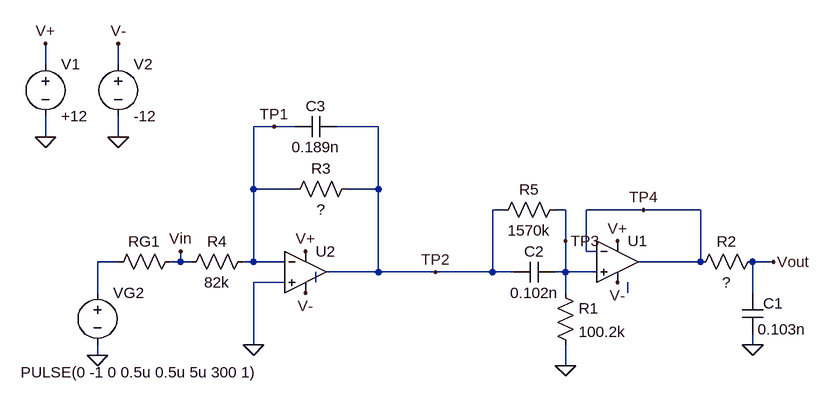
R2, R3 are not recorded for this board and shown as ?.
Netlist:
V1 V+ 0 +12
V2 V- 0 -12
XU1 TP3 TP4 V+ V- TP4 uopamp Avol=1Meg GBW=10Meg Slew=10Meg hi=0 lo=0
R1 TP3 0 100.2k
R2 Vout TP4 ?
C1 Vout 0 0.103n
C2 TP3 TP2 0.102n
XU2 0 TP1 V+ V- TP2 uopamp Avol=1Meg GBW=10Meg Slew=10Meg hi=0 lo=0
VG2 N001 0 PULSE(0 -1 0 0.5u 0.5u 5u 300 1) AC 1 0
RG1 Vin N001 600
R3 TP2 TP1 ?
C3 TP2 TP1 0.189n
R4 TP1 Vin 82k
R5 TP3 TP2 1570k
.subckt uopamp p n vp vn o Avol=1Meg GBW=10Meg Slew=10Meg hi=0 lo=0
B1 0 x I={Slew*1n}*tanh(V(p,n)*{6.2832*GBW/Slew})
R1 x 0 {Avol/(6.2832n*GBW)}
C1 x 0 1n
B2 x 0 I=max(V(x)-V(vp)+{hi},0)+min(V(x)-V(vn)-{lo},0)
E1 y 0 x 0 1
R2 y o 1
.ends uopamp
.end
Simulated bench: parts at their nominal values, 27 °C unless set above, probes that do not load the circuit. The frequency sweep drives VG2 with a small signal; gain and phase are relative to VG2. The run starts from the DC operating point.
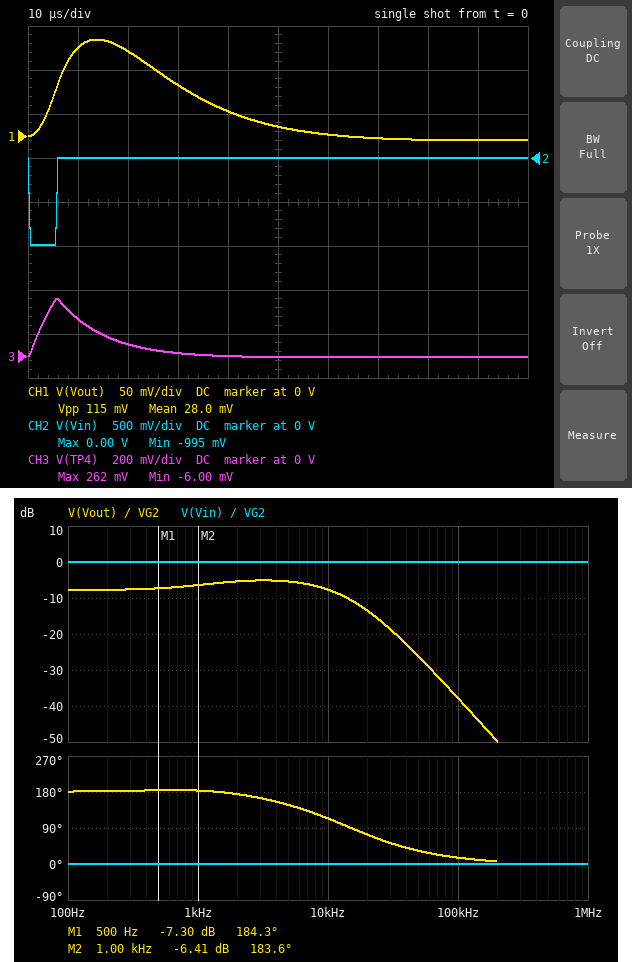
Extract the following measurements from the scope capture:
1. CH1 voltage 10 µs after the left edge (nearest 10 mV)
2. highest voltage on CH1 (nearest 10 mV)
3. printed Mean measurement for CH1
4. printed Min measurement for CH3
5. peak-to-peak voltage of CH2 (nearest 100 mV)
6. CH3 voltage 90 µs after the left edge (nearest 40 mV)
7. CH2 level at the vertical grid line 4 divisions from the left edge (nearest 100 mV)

100 mV
110 mV
28.0 mV
-6.00 mV
1.0 V
0 V
0 V
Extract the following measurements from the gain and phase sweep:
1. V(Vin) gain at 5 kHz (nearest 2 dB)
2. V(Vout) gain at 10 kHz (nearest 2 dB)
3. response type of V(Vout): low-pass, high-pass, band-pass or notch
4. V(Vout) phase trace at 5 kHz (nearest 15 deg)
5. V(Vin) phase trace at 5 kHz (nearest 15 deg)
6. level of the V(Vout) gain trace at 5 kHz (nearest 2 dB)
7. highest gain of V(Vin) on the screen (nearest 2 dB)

0 dB
-8 dB
low-pass
150 deg
0 deg
-6 dB
0 dB
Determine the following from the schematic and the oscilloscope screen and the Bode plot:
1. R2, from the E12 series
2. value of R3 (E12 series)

120 kΩ
560 kΩ
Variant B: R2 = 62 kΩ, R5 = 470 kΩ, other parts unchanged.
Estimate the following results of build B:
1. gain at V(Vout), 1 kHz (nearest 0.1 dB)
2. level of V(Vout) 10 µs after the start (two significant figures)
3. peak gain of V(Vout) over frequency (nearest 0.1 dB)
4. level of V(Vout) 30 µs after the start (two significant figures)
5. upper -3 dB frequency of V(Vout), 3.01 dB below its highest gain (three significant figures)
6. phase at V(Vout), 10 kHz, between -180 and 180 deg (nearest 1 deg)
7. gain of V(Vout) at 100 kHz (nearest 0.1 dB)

0.3 dB
150 mV
1.5 dB
64 mV
1.91 kHz
120 deg
-32.3 dB
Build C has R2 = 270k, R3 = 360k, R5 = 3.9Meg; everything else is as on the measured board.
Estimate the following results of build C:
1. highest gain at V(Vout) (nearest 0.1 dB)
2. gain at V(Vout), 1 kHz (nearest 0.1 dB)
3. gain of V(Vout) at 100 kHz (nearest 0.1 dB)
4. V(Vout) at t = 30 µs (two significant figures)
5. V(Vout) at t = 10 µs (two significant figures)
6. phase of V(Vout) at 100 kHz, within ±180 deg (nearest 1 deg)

-7.0 dB
-11.5 dB
-44.8 dB
45 mV
52 mV
12 deg
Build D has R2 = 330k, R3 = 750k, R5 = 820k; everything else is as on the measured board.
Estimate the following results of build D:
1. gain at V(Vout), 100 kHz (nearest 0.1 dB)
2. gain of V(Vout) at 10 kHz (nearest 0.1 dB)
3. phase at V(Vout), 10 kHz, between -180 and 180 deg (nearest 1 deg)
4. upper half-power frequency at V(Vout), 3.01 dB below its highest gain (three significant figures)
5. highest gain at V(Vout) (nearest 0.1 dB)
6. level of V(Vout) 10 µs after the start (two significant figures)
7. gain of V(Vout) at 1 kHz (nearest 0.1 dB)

-46.6 dB
-13.3 dB
81 deg
1.60 kHz
-0.1 dB
45 mV
-1.8 dB
